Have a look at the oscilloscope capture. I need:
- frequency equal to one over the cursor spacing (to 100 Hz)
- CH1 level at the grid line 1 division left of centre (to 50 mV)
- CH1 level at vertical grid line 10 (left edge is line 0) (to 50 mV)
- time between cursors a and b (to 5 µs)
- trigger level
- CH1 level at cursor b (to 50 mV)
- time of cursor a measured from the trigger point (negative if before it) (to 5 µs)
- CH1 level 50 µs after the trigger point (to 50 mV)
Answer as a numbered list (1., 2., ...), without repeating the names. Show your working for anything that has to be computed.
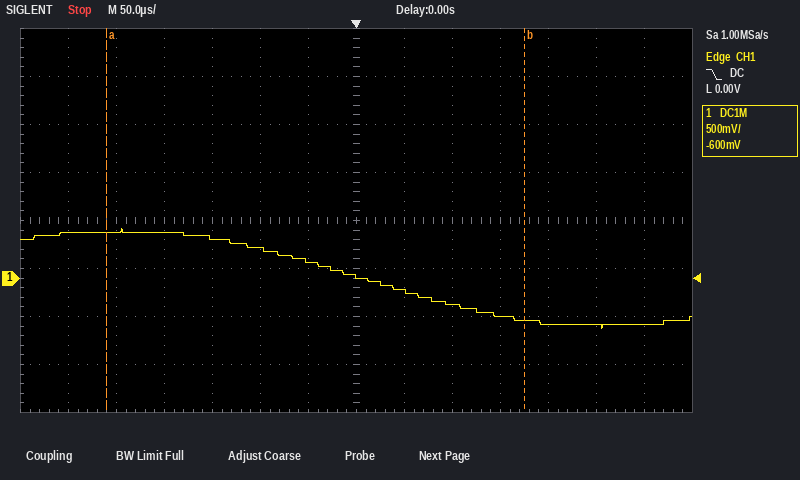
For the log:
1. 1 / 435 µs ≈ 2.3 kHz
2. 150 mV
3. -400 mV
4. 435 µs
5. 0.00 V
6. -450 mV
7. -260 µs
8. -150 mV
